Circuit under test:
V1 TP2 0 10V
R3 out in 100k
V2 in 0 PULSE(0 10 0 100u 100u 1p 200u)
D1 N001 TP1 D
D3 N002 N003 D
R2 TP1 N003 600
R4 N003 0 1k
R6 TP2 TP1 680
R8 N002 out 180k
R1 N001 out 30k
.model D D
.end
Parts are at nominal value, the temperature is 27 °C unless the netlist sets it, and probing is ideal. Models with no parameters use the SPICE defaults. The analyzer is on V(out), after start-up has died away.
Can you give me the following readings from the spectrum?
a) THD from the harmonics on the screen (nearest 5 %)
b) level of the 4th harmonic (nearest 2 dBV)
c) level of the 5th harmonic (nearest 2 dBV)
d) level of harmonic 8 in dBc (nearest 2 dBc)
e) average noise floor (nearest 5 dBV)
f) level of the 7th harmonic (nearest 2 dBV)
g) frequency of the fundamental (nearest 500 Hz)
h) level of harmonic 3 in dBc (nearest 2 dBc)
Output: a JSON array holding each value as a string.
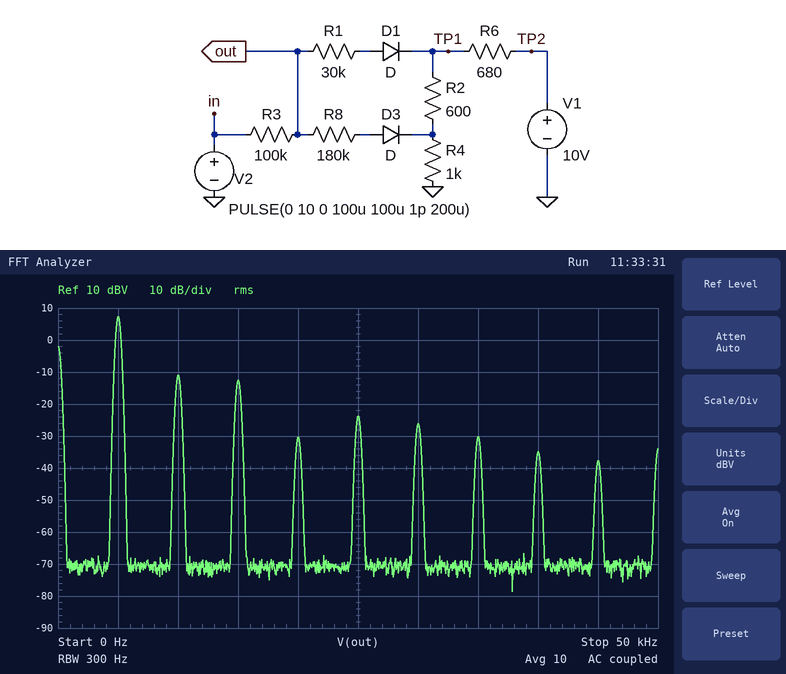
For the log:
["15 %", "-30 dBV", "-24 dBV", "-42 dBc", "-70 dBV", "-30 dBV", "5.0 kHz", "-20 dBc"]
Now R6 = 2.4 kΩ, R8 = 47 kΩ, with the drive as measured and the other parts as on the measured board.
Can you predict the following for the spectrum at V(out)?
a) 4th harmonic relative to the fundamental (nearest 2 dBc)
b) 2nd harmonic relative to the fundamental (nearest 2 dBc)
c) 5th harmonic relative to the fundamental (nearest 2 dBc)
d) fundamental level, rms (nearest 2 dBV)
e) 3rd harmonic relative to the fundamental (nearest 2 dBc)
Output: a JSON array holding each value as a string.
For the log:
["-20 dBc", "-10 dBc", "-26 dBc", "2 dBV", "-14 dBc"]
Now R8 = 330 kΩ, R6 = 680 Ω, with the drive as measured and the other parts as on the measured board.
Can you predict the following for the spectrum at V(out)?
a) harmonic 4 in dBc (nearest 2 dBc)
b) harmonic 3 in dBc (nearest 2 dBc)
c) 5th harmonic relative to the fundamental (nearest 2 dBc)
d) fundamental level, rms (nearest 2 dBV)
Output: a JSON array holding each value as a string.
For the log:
["-30 dBc", "-22 dBc", "-36 dBc", "8 dBV"]
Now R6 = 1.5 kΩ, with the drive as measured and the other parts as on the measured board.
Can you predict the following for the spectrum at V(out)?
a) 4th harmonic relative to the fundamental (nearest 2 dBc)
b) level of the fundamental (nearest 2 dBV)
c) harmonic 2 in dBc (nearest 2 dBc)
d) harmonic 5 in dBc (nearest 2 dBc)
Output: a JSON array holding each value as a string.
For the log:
["-26 dBc", "6 dBV", "-12 dBc", "-30 dBc"]
